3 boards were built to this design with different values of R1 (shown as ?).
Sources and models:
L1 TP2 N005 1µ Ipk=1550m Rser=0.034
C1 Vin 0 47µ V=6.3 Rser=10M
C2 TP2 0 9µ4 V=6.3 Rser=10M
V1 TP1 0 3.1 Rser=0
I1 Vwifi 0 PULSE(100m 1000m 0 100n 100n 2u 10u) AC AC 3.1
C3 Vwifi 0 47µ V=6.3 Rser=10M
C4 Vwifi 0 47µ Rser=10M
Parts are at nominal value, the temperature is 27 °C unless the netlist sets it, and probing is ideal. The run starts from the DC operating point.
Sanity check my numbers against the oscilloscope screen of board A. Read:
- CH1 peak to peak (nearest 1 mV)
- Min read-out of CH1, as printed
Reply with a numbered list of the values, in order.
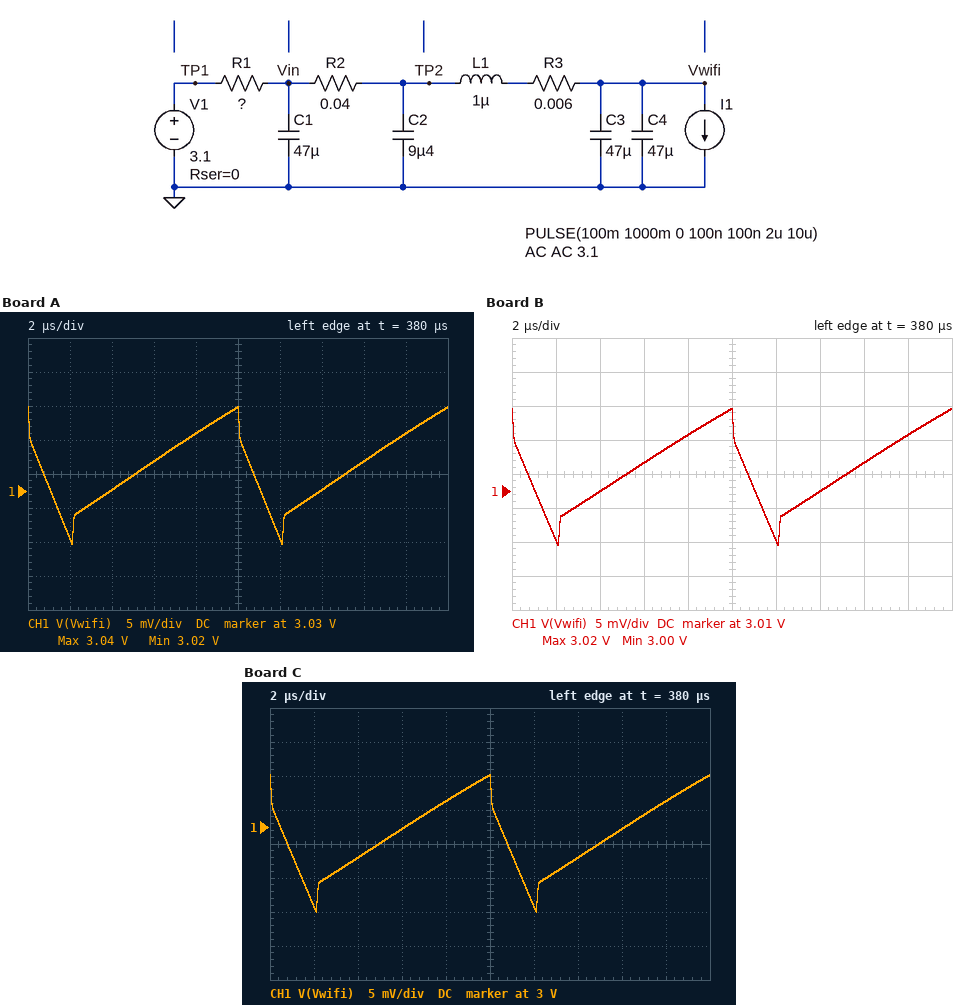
1. 20 mV
2. 3.02 V
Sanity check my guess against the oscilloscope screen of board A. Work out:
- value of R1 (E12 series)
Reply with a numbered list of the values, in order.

1. 0.15 Ω
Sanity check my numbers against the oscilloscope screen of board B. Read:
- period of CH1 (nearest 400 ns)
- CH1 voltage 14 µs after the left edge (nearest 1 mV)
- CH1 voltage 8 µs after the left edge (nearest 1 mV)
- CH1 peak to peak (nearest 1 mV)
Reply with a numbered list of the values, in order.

1. 10.0 µs
2. 3.010 V
3. 3.018 V
4. 20 mV
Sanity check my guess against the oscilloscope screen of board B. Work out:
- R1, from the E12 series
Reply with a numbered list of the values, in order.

1. 0.22 Ω
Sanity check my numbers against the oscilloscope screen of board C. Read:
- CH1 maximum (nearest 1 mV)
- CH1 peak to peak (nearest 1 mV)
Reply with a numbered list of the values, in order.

1. 3.008 V
2. 20 mV
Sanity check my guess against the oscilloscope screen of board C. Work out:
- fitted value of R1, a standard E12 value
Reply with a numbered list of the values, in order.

1. 0.27 Ω
